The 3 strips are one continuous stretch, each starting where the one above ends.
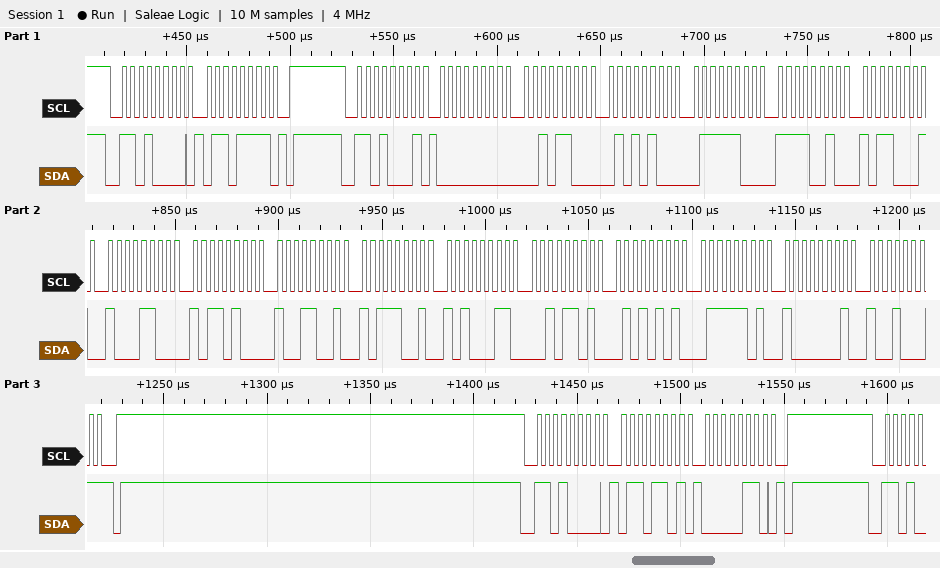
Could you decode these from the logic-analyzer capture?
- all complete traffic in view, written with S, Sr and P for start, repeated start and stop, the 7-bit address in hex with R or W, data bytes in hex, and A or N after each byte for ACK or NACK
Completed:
S 68W A 6F A P S 68R A 00 A 2C A 54 A 7C A F2 A B1 A 8C A B4 A 99 A B9 A A3 A 2D A 55 A 7D A 81 A 91 N P S 68W A 6D A 06 A P
